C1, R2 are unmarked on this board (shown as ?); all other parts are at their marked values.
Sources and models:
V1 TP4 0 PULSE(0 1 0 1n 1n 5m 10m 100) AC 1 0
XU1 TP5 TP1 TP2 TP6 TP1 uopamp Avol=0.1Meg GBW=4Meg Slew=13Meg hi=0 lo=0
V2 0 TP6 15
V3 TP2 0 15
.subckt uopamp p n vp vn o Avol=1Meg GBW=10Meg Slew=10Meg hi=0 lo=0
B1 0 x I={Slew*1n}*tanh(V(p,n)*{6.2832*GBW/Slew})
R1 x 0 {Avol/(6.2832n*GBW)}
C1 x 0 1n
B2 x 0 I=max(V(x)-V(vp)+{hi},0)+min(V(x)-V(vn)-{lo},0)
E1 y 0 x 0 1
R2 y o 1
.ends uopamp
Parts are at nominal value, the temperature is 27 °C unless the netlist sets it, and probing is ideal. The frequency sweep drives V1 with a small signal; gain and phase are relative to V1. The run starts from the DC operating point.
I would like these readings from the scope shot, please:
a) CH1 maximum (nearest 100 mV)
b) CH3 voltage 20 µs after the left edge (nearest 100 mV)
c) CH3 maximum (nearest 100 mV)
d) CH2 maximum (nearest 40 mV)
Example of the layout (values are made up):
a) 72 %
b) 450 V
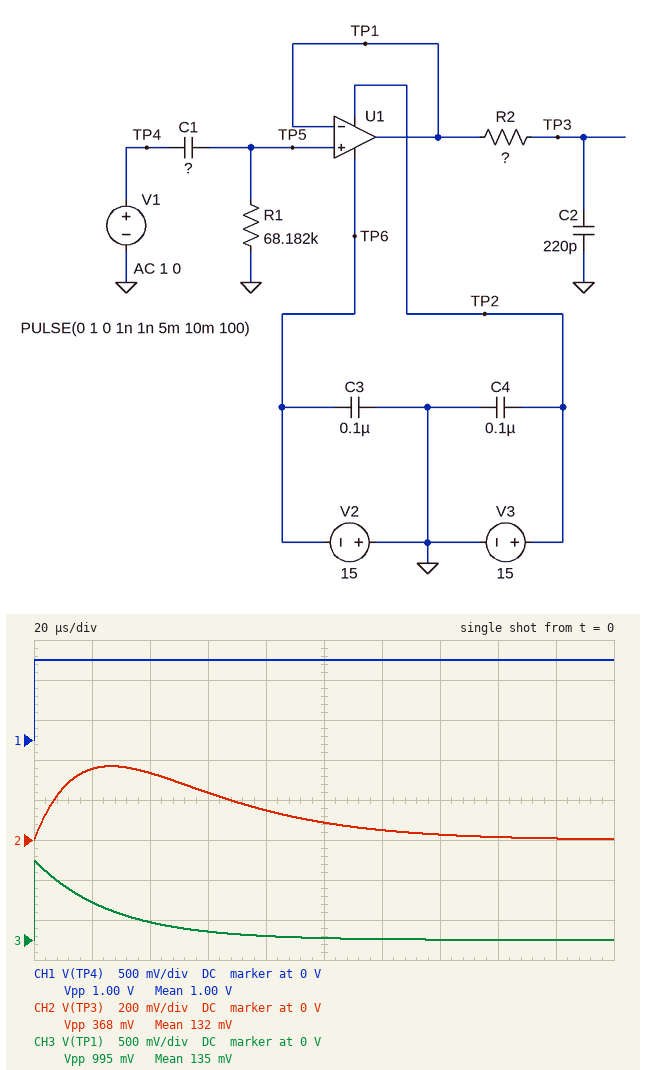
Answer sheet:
a) 1.0 V
b) 500 mV
c) 1.0 V
d) 360 mV
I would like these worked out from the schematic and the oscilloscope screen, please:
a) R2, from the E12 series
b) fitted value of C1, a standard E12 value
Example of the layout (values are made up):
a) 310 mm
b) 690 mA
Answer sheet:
a) 120 kΩ
b) 390 pF
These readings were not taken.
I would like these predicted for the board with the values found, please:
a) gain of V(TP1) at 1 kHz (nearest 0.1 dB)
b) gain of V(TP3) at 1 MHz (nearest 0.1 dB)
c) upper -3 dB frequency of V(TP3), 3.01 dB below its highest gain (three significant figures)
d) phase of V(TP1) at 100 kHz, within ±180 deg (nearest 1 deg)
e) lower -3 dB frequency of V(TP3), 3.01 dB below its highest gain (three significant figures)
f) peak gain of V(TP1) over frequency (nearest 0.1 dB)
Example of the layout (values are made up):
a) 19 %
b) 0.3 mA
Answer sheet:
a) -15.7 dB
b) -44.7 dB
c) 14.5 kHz
d) 2 deg
e) 2.49 kHz
f) 0 dB
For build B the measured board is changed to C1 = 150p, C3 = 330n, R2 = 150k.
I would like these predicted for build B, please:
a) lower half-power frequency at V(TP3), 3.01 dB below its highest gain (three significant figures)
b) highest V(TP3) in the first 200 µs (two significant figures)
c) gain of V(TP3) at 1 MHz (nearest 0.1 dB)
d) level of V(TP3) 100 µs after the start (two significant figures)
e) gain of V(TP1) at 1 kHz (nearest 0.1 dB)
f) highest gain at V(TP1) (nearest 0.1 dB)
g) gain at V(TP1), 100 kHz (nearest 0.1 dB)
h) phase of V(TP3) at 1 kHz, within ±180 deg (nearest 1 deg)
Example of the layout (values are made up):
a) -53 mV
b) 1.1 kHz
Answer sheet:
a) 3.18 kHz
b) 180 mV
c) -46.6 dB
d) 22 mV
e) -23.9 dB
f) 0 dB
g) -0.1 dB
h) 75 deg
